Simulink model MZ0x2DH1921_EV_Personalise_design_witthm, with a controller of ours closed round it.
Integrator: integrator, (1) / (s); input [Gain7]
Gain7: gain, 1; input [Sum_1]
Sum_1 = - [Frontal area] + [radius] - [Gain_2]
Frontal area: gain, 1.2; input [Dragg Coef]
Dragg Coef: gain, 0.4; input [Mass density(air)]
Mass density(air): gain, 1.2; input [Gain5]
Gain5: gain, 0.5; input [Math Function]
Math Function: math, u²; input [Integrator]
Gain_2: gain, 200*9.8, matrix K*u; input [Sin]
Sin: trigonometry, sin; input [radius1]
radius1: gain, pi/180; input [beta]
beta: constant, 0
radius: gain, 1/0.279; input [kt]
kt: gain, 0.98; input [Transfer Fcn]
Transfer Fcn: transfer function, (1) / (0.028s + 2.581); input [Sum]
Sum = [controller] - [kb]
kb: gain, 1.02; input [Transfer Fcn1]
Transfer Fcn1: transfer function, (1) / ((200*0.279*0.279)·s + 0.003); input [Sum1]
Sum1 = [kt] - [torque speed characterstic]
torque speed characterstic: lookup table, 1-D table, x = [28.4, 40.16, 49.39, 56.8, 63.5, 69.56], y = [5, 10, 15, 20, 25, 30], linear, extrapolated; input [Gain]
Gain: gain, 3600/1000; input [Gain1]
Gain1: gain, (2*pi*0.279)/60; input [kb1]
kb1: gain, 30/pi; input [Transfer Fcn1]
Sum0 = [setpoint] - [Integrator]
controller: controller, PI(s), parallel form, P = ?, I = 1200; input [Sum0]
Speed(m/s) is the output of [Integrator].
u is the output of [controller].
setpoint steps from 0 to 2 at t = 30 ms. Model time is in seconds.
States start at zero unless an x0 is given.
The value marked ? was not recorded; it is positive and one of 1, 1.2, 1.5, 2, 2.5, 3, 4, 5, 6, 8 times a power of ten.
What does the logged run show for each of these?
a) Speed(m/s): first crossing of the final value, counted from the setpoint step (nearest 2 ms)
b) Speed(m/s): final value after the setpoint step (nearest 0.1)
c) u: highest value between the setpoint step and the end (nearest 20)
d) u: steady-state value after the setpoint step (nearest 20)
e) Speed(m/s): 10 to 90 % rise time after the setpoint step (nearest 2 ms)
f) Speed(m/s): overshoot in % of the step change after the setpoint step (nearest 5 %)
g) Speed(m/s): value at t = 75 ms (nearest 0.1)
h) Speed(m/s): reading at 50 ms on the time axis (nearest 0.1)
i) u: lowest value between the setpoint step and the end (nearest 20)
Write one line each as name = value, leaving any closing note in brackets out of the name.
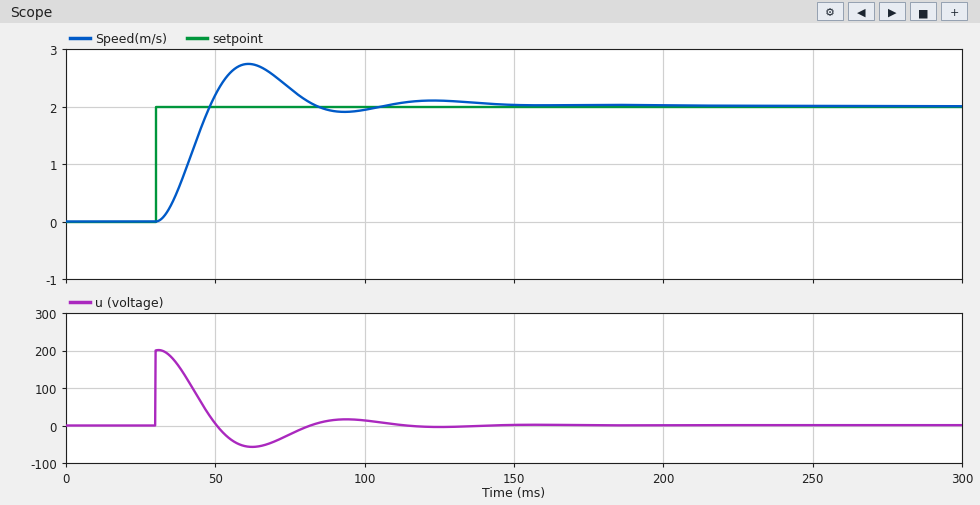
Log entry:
Speed(m/s): first crossing of the final value, counted from the setpoint step = 18 ms
Speed(m/s): final value after the setpoint step = 2.0
u: highest value between the setpoint step and the end = 200
u: steady-state value after the setpoint step = 0
Speed(m/s): 10 to 90 % rise time after the setpoint step = 12 ms
Speed(m/s): overshoot in % of the step change after the setpoint step = 35 %
Speed(m/s): value at t = 75 ms = 2.3
Speed(m/s): reading at 50 ms on the time axis = 2.2
u: lowest value between the setpoint step and the end = -60
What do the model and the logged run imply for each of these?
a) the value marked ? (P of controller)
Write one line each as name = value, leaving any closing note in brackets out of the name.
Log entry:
the value marked ? = 100
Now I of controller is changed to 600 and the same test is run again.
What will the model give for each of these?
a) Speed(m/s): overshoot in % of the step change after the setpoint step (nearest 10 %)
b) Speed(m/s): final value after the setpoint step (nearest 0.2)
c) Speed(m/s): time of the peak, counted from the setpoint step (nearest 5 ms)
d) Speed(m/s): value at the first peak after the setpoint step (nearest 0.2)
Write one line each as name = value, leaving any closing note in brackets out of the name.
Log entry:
Speed(m/s): overshoot in % of the step change after the setpoint step = 30 %
Speed(m/s): final value after the setpoint step = 2.0
Speed(m/s): time of the peak, counted from the setpoint step = 30 ms
Speed(m/s): value at the first peak after the setpoint step = 2.6
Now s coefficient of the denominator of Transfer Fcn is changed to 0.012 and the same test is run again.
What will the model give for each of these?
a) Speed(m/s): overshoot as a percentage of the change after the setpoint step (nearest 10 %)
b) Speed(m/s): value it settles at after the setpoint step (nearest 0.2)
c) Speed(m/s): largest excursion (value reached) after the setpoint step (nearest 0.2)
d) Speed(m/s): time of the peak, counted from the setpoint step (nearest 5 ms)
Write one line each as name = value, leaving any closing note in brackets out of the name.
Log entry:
Speed(m/s): overshoot as a percentage of the change after the setpoint step = 20 %
Speed(m/s): value it settles at after the setpoint step = 2.0
Speed(m/s): largest excursion (value reached) after the setpoint step = 2.4
Speed(m/s): time of the peak, counted from the setpoint step = 25 ms
